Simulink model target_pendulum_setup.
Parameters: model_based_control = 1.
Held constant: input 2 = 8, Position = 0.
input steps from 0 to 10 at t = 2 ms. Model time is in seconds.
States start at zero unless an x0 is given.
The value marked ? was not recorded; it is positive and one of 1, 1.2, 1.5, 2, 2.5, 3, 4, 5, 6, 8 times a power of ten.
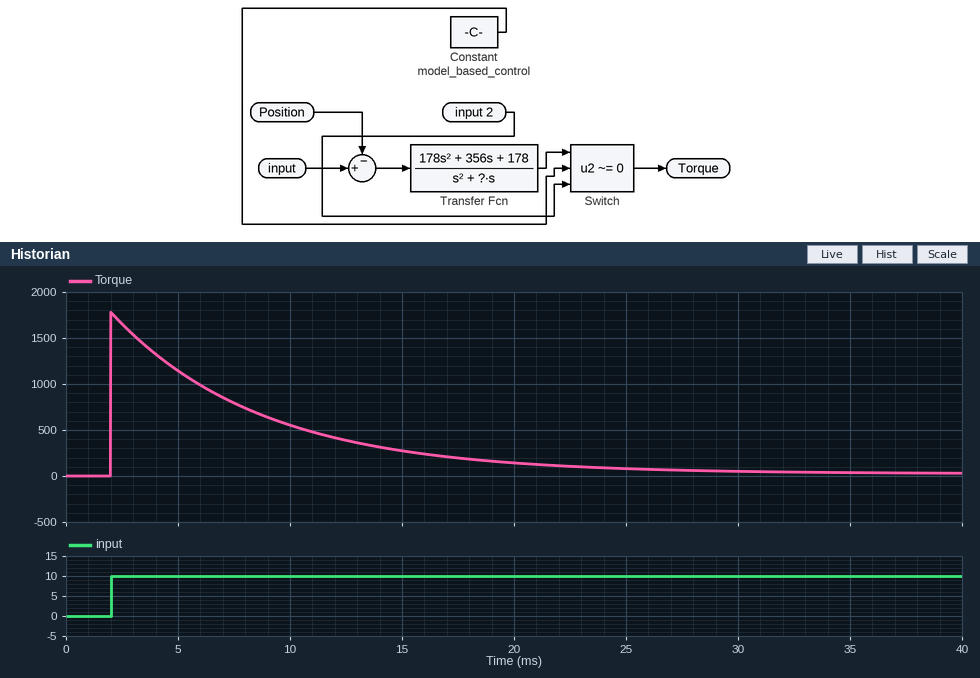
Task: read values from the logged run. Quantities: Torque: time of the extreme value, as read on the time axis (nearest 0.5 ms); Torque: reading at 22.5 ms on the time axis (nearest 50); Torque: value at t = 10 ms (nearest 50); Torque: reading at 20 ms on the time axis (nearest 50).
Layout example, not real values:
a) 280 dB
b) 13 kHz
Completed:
a) 2.0 ms
b) 100
c) 550
d) 150
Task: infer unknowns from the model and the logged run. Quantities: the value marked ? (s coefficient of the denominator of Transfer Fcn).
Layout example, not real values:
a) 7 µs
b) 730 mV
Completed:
a) 150
